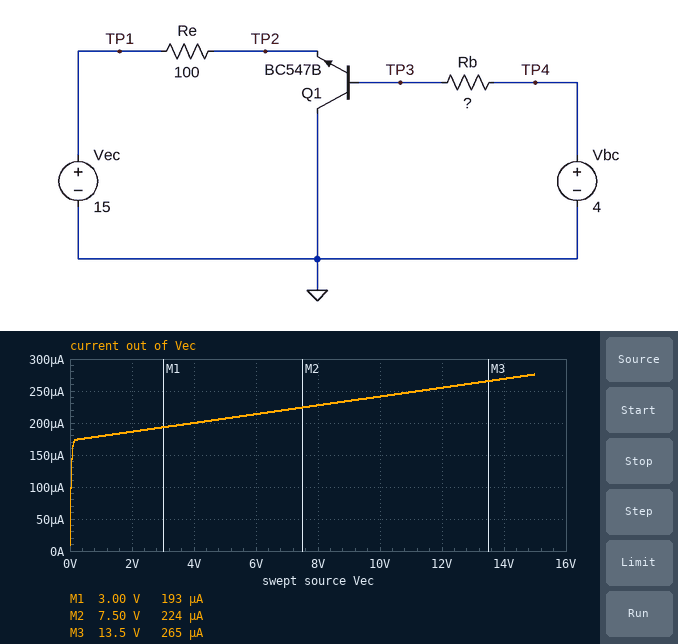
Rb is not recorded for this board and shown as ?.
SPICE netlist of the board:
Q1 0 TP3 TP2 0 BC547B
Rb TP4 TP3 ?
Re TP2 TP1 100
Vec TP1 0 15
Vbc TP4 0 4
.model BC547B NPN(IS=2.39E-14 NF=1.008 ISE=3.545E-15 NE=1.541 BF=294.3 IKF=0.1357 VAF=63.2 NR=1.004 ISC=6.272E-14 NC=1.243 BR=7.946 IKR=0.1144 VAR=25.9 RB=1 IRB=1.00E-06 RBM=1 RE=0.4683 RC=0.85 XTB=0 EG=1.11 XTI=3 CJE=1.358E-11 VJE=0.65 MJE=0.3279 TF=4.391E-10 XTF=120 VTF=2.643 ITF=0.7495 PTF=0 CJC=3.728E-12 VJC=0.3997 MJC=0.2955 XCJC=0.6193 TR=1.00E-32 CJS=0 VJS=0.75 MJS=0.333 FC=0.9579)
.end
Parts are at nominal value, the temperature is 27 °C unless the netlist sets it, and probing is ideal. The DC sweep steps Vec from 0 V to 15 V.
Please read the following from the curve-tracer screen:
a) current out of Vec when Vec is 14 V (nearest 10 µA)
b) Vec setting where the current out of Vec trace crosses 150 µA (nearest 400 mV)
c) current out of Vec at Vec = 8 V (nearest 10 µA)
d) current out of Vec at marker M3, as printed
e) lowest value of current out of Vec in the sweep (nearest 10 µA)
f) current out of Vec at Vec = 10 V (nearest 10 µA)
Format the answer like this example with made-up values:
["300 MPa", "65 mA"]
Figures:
["270 µA", "0 V", "230 µA", "265 µA", "10 µA", "240 µA"]
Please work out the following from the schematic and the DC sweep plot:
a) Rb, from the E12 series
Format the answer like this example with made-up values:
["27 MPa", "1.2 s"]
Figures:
["120 kΩ"]
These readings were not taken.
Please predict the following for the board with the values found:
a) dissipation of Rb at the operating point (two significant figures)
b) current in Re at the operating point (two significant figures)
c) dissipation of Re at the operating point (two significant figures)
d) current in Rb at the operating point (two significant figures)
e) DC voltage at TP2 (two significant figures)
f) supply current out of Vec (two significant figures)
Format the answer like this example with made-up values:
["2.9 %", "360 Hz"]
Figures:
["97 µW", "280 µA", "7.6 µW", "28 µA", "15 V", "280 µA"]
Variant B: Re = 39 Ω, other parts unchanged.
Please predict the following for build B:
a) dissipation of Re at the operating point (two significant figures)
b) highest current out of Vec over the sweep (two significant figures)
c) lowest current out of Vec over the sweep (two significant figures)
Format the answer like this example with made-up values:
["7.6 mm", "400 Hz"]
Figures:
["3.0 µW", "280 µA", "11 µA"]
